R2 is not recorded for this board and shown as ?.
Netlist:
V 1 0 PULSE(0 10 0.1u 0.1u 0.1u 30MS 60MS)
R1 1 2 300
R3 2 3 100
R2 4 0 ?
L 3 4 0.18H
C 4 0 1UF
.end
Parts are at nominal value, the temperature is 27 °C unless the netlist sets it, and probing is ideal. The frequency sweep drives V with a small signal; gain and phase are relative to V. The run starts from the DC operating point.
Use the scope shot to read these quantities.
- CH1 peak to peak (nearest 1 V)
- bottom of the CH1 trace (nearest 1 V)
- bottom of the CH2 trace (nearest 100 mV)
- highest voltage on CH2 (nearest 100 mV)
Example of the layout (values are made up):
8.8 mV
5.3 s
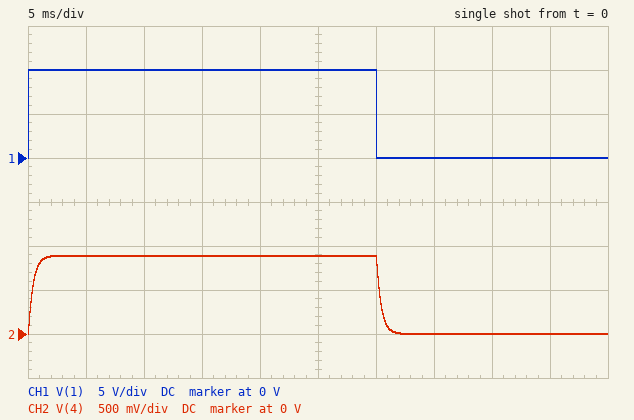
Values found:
10 V
0 V
0 V
900 mV
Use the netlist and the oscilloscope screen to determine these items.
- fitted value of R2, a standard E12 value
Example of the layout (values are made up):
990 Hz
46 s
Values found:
39 Ω
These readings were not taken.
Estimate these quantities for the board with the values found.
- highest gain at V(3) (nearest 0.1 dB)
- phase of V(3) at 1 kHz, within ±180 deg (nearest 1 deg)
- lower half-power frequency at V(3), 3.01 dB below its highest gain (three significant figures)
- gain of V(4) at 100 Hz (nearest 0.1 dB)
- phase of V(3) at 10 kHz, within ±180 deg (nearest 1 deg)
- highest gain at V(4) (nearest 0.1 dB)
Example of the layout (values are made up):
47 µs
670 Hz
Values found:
0 dB
19 deg
388 Hz
-21.3 dB
2 deg
-21.0 dB
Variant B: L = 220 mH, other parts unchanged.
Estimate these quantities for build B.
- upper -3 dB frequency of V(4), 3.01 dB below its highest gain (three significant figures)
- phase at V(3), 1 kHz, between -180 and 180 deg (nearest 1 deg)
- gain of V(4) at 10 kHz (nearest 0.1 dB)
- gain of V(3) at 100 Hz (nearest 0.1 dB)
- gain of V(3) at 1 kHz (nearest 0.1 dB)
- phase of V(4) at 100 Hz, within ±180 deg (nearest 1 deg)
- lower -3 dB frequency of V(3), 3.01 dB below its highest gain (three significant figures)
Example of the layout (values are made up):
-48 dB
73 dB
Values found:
318 Hz
16 deg
-59.4 dB
-10.2 dB
-0.4 dB
-19 deg
317 Hz
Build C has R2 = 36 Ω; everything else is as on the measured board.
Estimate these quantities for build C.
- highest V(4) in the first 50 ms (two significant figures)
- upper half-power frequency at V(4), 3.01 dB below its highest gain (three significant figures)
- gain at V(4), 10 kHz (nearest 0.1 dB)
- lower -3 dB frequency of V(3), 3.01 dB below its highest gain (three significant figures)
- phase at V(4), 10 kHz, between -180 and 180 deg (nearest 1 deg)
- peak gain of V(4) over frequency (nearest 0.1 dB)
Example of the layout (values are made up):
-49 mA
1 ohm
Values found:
830 mV
386 Hz
-57.8 dB
385 Hz
-154 deg
-21.7 dB
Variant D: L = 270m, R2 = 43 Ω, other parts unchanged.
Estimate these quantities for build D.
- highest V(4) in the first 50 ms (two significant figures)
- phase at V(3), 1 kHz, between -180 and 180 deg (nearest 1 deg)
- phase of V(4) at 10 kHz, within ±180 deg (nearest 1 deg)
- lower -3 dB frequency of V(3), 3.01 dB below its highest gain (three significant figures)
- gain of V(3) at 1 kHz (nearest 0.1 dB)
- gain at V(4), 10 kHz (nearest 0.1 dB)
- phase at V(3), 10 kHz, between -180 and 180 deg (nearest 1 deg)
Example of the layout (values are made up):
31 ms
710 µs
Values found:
970 mV
13 deg
-158 deg
260 Hz
-0.3 dB
-61.1 dB
1 deg
